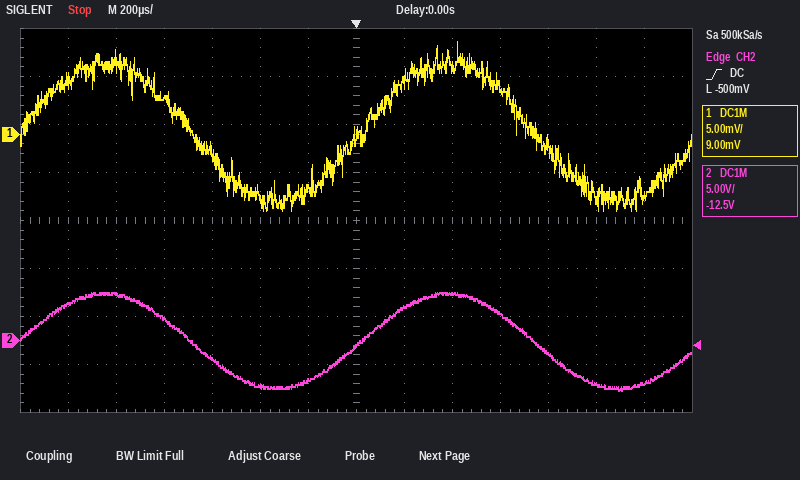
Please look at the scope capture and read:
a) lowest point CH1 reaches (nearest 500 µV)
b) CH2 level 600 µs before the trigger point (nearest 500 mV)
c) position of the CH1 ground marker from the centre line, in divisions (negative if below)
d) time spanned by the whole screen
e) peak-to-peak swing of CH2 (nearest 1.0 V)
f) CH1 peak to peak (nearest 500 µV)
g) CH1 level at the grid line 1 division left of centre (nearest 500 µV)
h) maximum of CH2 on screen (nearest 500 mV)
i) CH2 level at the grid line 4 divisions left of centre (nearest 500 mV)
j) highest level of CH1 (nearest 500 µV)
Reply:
-8.0 mV
-2.0 V
+1.8 div
2.8 ms
10.0 V
17.5 mV
-5.5 mV
5.0 V
2.5 V
9.5 mV
